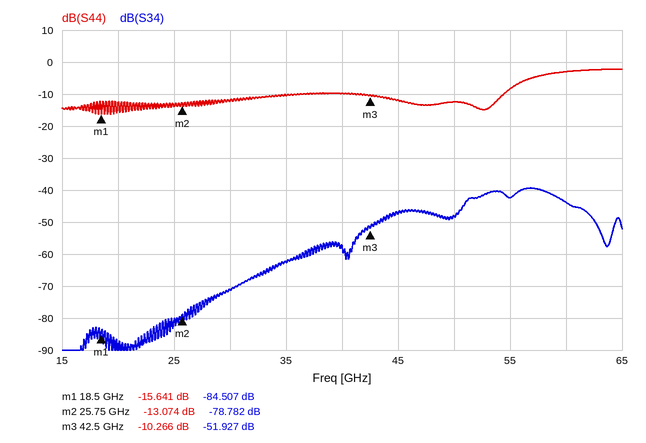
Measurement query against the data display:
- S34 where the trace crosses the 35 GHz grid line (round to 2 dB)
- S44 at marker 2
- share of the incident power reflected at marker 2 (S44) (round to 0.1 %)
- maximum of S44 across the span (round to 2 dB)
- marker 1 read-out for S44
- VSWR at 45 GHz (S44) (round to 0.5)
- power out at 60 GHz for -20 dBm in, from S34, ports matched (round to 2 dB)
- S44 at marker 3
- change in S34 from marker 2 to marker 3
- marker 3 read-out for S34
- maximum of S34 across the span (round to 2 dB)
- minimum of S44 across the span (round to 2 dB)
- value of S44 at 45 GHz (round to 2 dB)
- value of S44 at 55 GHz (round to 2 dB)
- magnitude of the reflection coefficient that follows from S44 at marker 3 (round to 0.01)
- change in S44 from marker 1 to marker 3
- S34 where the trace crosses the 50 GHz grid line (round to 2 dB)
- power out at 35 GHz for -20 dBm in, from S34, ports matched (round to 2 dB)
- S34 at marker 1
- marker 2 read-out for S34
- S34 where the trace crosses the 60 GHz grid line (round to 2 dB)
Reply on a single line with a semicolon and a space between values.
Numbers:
-62 dB; -13.074 dB; 4.9 %; -2 dB; -15.641 dB; 1.5; -64 dBm; -10.266 dB; 26.855 dB; -51.927 dB; -40 dB; -16 dB; -12 dB; -8 dB; 0.31; 5.375 dB; -48 dB; -82 dBm; -84.507 dB; -78.782 dB; -44 dB
